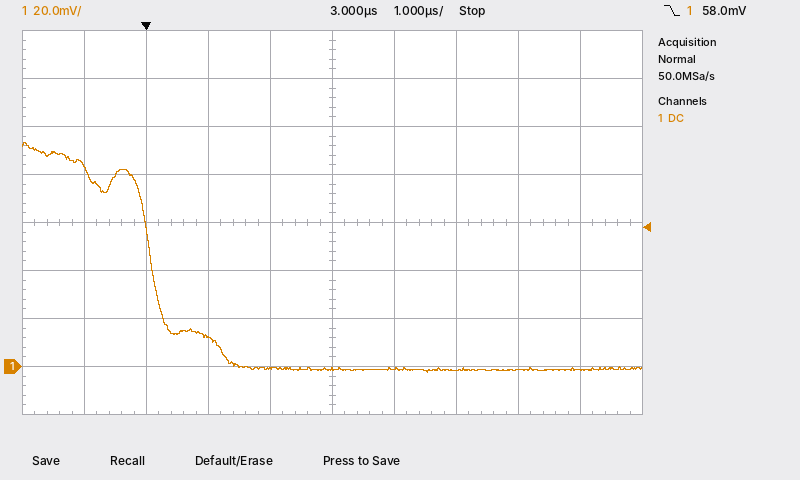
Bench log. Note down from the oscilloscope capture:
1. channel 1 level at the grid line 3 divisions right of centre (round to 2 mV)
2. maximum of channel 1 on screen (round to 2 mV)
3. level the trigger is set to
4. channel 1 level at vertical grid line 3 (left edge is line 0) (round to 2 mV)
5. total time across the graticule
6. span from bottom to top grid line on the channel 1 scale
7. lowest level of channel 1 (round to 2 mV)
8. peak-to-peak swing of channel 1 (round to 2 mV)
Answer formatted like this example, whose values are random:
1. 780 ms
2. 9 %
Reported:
1. -2 mV
2. 94 mV
3. 58.0 mV
4. 12 mV
5. 10 µs
6. 160 mV
7. -2 mV
8. 96 mV
